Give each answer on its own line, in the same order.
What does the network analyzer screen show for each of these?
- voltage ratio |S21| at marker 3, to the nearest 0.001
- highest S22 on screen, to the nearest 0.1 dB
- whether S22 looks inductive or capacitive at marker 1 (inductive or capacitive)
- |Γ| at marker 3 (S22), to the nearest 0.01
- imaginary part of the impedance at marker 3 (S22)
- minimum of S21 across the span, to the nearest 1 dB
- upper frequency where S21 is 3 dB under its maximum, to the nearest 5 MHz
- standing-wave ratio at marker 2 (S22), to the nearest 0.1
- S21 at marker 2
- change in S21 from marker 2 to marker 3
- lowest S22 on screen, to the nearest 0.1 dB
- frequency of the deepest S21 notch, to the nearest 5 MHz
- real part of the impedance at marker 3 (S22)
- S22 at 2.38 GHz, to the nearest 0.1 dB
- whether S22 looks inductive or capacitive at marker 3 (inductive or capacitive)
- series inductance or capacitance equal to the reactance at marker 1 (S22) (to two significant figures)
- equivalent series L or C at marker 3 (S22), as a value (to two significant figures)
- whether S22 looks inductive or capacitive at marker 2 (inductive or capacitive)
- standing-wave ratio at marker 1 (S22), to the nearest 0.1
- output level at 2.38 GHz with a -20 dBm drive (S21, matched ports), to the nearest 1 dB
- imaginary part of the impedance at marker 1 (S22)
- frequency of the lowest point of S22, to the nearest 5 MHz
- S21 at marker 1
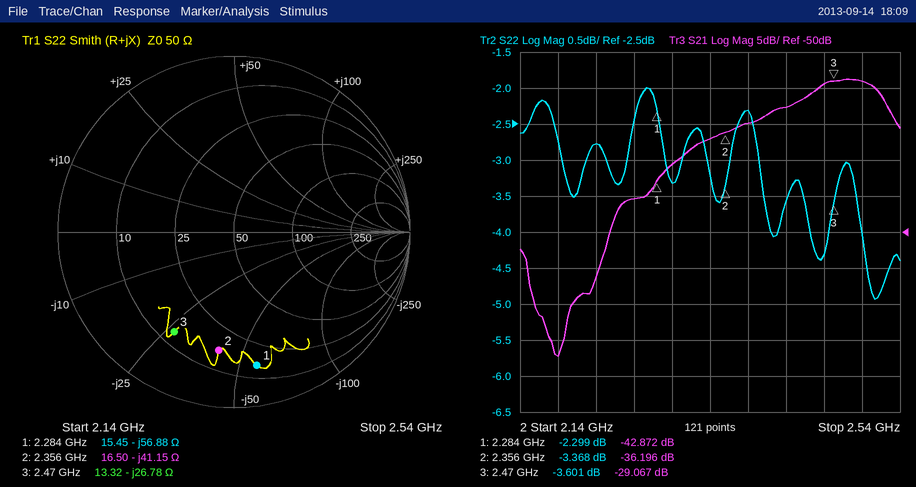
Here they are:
0.035
-2.0 dB
capacitive
0.66
-26.78 Ω
-67 dB
2.525 GHz
5.2
-36.196 dB
7.129 dB
-4.9 dB
2.180 GHz
13.32 Ω
-2.3 dB
capacitive
1.2 pF
2.4 pF
capacitive
7.6
-55 dBm
-56.88 Ω
2.515 GHz
-42.872 dB
